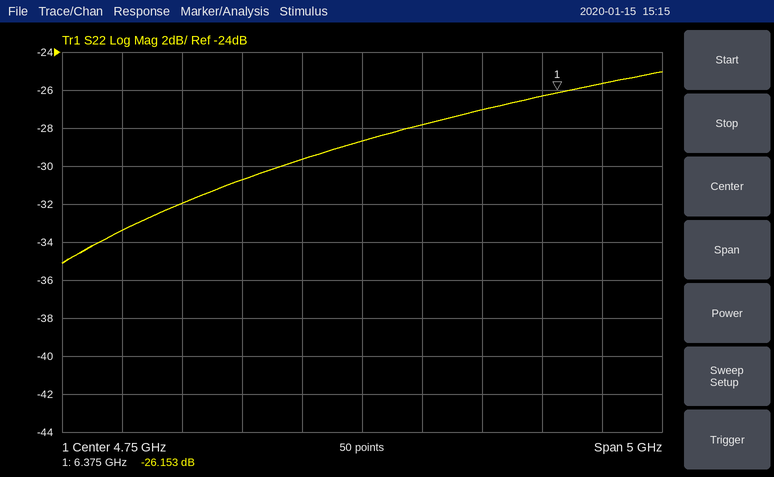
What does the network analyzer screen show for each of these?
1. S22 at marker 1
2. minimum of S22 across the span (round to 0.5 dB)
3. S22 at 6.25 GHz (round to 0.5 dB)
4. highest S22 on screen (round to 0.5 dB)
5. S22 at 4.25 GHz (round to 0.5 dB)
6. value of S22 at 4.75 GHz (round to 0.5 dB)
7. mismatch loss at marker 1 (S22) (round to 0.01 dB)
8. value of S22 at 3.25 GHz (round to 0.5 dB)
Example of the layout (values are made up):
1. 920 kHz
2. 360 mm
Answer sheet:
1. -26.153 dB
2. -35.0 dB
3. -26.5 dB
4. -25.0 dB
5. -29.5 dB
6. -28.5 dB
7. 0.01 dB
8. -32.0 dB
